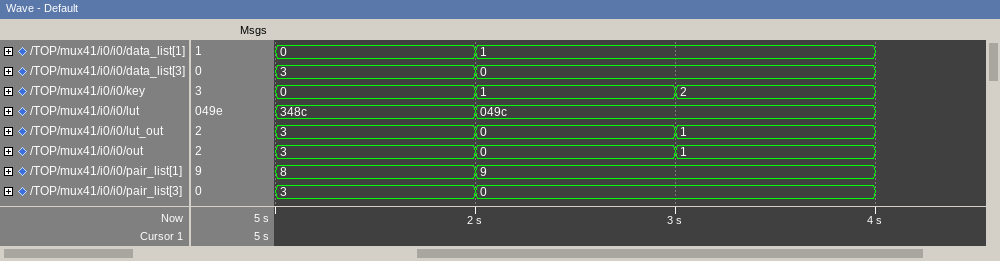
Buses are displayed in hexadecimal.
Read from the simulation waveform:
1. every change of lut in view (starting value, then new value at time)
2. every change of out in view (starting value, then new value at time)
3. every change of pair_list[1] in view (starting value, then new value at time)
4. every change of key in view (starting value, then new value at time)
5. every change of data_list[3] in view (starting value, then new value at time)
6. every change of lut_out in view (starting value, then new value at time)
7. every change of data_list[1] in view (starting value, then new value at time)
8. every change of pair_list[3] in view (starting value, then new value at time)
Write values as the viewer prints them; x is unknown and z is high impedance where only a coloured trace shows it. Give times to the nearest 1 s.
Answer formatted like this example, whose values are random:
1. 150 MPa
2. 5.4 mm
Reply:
1. 348c, 049c at 2 s
2. 3, 0 at 2 s, 1 at 3 s
3. 8, 9 at 2 s
4. 0, 1 at 2 s, 2 at 3 s
5. 3, 0 at 2 s
6. 3, 0 at 2 s, 1 at 3 s
7. 0, 1 at 2 s
8. 3, 0 at 2 s
